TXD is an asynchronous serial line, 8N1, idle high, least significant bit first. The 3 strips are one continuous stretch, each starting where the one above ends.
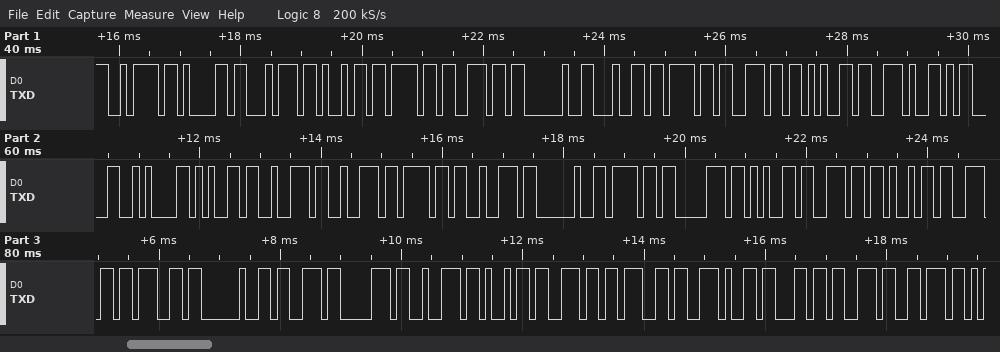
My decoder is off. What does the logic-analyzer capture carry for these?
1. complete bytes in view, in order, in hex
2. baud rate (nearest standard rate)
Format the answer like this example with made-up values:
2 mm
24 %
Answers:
7A 61 74 69 6F 6E 20 64 6F 6E 65 2E 0D 0A 65 72 72 6F 72 20 6F 70 65 6E 69 6E 67 20 73 70 72 69 6E 67 2E 63 73 76
9600 baud
